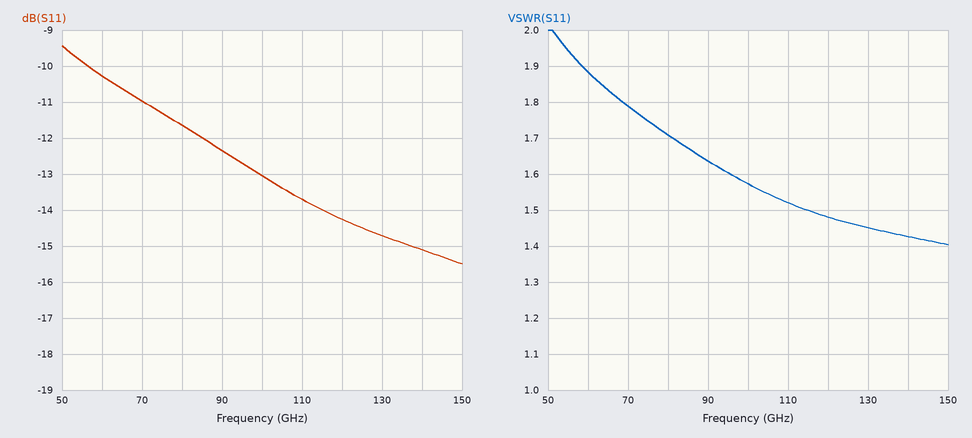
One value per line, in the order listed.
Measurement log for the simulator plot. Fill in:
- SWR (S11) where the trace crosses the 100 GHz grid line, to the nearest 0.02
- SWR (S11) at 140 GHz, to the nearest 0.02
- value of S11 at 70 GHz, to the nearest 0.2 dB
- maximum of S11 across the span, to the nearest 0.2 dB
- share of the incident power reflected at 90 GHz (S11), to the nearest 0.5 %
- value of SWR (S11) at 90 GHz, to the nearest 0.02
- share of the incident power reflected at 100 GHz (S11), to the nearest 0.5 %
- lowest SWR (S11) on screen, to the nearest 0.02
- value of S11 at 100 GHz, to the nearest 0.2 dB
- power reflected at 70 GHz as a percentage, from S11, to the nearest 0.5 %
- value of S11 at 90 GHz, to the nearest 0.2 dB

1.58
1.42
-11.0 dB
-9.4 dB
6.0 %
1.64
5.0 %
1.40
-13.0 dB
8.0 %
-12.4 dB
